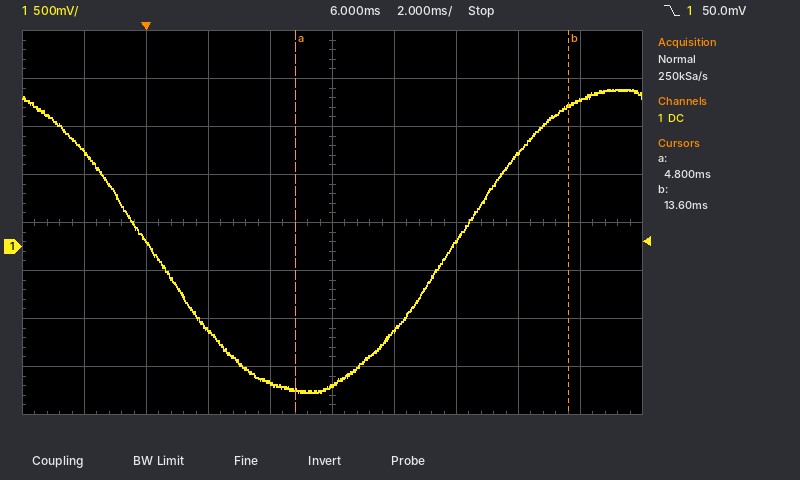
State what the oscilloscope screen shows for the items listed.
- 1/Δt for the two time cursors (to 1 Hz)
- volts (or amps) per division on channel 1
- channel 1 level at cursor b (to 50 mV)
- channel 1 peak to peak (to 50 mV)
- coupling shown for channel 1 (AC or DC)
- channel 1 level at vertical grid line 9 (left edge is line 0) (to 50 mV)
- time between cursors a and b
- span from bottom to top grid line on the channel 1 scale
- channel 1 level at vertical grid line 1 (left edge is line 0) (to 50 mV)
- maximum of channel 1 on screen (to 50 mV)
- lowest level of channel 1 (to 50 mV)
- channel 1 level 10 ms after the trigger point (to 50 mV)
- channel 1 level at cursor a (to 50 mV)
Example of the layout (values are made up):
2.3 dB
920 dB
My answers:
114 Hz
500 mV
1.45 V
3.15 V
DC
1.50 V
8.8 ms
4 V
1.00 V
1.65 V
-1.50 V
50 mV
-1.50 V
